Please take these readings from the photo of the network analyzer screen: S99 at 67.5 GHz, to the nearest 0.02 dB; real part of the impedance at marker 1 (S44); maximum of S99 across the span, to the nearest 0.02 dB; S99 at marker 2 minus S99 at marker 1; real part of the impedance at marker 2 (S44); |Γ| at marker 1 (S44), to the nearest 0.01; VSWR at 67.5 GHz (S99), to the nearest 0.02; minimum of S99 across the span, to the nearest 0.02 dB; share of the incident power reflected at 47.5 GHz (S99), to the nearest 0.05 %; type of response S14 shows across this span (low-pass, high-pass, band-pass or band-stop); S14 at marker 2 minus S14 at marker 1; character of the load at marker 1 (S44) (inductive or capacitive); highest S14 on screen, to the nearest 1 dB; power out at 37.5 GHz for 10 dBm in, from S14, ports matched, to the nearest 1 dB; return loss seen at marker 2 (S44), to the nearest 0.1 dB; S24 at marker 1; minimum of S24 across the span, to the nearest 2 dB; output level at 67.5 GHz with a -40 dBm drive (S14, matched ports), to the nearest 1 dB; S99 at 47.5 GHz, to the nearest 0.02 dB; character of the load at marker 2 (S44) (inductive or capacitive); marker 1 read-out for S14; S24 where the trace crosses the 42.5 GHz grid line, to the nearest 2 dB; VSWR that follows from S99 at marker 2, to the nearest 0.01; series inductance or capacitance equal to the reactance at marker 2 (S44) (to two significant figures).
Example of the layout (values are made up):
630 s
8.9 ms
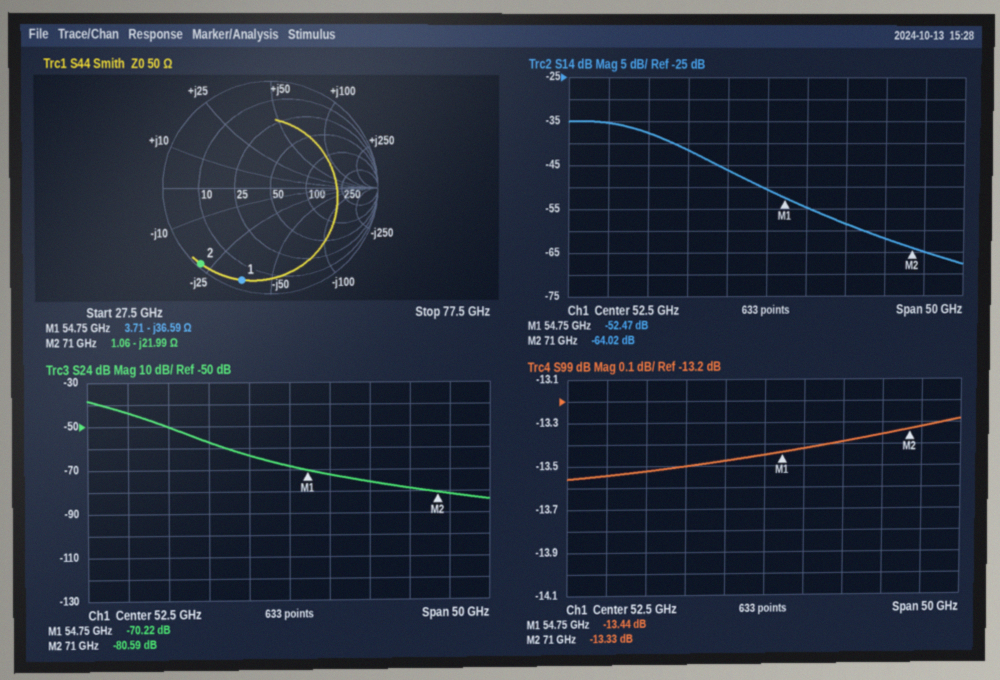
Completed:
-13.36 dB
3.71 Ω
-13.28 dB
0.11 dB
1.06 Ω
0.91
1.54
-13.56 dB
4.50 %
low-pass
-11.55 dB
capacitive
-35 dB
-28 dBm
0.3 dB
-70.22 dB
-84 dB
-102 dBm
-13.48 dB
capacitive
-52.47 dB
-58 dB
1.55
100 fF
